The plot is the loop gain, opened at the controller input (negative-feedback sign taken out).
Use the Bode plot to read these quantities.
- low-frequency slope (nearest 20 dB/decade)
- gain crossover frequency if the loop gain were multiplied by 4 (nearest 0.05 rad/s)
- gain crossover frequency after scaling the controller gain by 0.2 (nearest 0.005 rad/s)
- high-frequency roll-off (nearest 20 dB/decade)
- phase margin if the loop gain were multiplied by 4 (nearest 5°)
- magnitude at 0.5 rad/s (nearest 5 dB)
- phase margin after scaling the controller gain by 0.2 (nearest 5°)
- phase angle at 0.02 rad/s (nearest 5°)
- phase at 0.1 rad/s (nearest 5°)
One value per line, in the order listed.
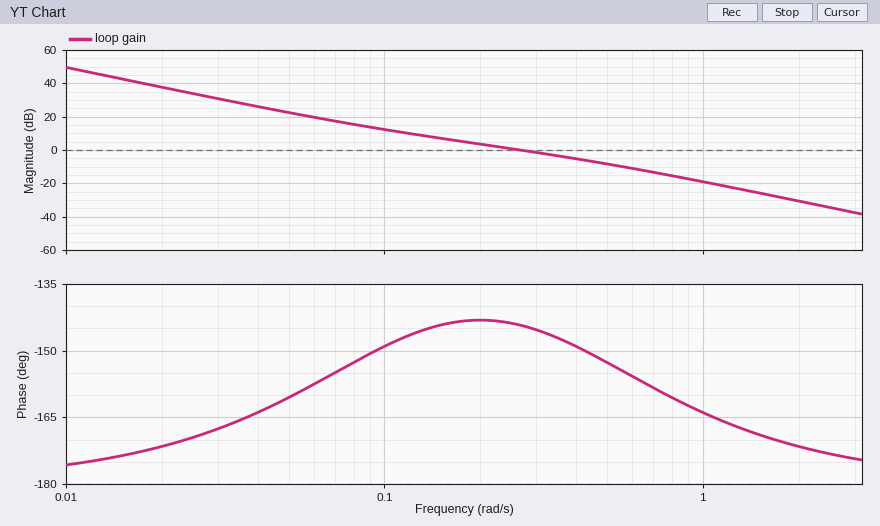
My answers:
-40 dB/decade
0.65 rad/s
0.090 rad/s
-40 dB/decade
25°
-10 dB
30°
-170°
-150°
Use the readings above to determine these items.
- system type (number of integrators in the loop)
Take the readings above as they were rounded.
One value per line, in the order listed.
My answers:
2
